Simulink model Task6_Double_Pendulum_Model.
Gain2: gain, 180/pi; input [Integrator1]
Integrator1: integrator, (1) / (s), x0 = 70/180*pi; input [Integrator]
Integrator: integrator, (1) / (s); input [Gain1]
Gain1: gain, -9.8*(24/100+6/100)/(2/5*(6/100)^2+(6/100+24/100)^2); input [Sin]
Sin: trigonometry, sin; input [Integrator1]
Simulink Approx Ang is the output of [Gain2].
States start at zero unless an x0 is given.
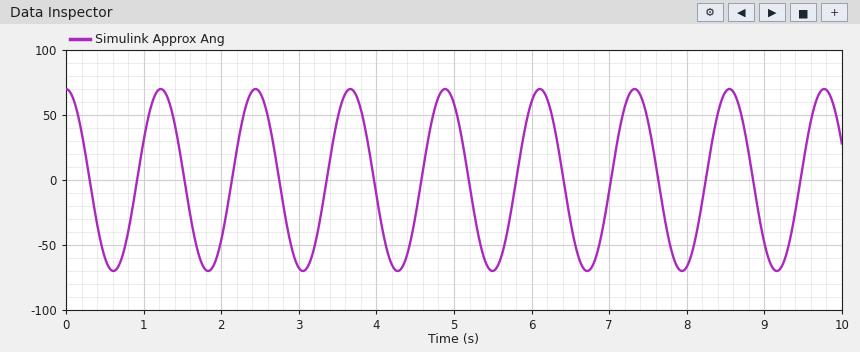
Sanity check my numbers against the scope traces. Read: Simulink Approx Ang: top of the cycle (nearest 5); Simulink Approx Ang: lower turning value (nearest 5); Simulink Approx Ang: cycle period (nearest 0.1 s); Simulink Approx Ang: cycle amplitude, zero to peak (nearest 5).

70
-70
1.2 s
70
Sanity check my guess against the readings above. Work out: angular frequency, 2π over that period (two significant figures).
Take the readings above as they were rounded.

5.2 rad/s
